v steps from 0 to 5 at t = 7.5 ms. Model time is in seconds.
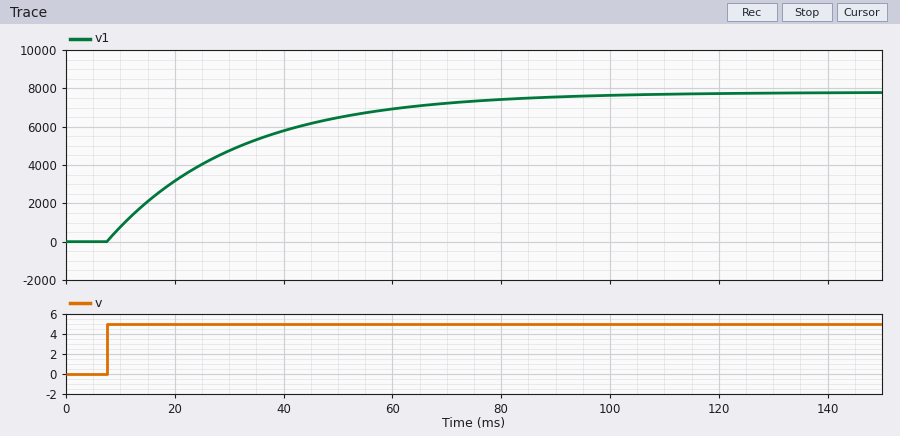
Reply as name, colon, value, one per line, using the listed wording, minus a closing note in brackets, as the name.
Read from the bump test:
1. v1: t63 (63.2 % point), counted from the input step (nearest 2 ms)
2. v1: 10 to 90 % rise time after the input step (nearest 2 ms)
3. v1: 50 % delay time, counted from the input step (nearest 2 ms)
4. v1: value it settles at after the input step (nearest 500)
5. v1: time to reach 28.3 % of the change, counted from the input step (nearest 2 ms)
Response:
v1: t63 (63.2 % point), counted from the input step: 24 ms
v1: 10 to 90 % rise time after the input step: 52 ms
v1: 50 % delay time, counted from the input step: 16 ms
v1: value it settles at after the input step: 8000
v1: time to reach 28.3 % of the change, counted from the input step: 8 ms
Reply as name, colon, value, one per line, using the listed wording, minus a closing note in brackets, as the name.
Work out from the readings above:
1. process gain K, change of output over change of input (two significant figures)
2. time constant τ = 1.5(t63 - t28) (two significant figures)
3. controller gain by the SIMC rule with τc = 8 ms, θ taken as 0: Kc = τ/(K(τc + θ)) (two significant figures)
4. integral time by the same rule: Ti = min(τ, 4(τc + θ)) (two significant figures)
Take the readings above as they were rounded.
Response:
process gain K, change of output over change of input: 1600
time constant τ = 1.5(t63 - t28): 24 ms
controller gain by the SIMC rule with τc = 8 ms, θ taken as 0: Kc = τ/(K(τc + θ)): 0.0019
integral time by the same rule: Ti = min(τ, 4(τc + θ)): 24 ms
